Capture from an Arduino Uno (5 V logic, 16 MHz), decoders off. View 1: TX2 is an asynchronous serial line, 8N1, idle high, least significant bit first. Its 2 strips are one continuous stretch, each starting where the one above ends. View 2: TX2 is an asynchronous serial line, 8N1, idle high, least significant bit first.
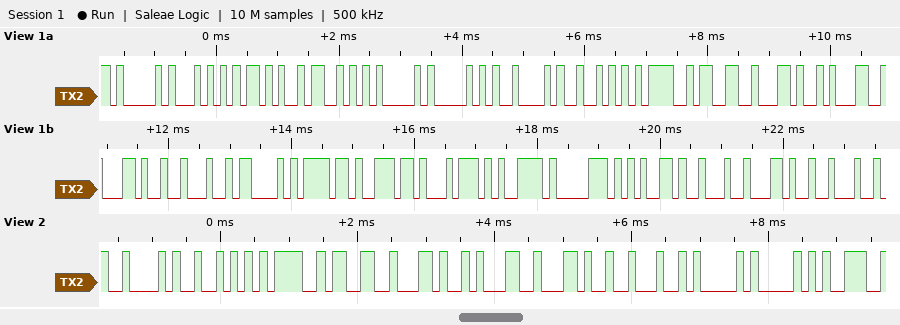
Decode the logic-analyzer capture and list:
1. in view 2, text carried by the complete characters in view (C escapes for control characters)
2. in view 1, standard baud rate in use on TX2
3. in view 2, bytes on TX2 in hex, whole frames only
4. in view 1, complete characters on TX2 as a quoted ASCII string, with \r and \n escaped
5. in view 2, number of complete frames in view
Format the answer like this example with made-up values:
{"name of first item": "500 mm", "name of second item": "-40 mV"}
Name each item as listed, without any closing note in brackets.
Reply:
{"in view 2, text carried by the complete characters in view": "\"BR=3,1,\\\"AP\"", "in view 1, standard baud rate in use on TX2": "9600 baud", "in view 2, bytes on TX2 in hex, whole frames only": "42 52 3D 33 2C 31 2C 22 41 50", "in view 1, complete characters on TX2 as a quoted ASCII string, with \\r and \\n escaped": "\"AT+SAPBR=3,1,\\\"Contype\\\",\\\"\"", "in view 2, number of complete frames in view": "10"}
